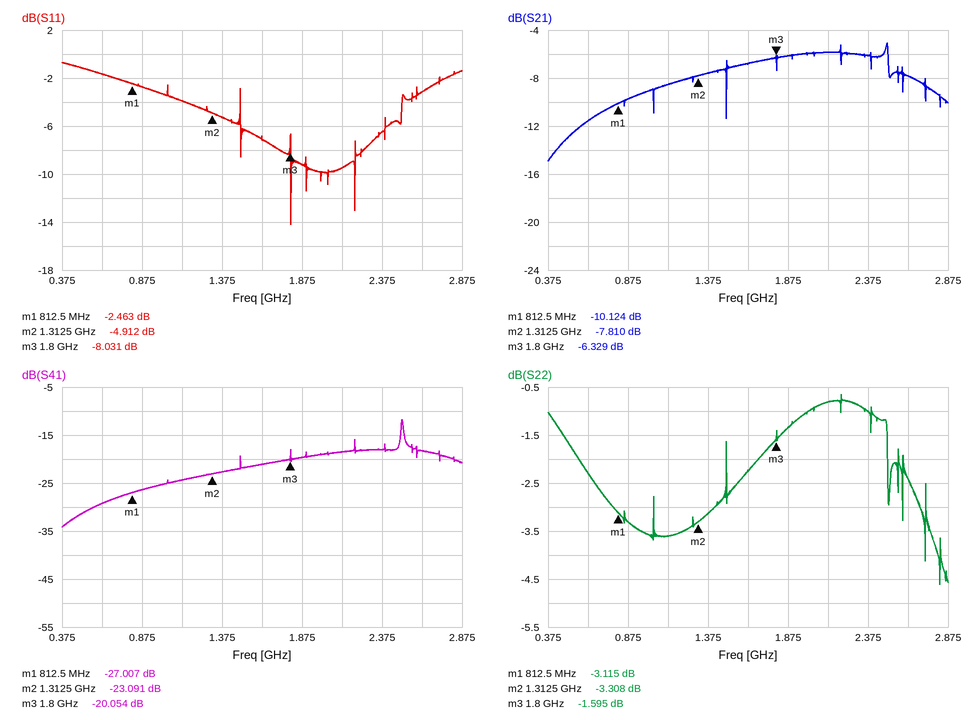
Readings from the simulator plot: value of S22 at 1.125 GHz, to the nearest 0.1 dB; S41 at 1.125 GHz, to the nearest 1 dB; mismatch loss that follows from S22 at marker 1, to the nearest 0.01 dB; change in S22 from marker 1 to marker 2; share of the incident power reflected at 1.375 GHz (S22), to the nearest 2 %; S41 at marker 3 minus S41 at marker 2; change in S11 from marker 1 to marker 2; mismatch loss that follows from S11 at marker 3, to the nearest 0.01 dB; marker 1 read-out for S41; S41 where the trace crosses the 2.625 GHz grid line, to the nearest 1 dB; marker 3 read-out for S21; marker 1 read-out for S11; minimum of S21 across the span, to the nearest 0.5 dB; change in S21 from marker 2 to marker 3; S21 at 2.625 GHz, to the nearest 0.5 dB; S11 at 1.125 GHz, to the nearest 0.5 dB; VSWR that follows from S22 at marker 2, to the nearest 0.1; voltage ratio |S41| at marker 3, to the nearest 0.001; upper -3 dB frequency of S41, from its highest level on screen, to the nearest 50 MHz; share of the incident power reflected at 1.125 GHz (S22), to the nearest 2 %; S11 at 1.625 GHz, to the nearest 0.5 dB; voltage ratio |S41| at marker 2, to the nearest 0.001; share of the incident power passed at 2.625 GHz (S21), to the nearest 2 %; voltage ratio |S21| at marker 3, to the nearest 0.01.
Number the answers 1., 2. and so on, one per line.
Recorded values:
1. -3.6 dB
2. -24 dB
3. 2.91 dB
4. -0.193 dB
5. 48 %
6. 3.037 dB
7. -2.449 dB
8. 0.74 dB
9. -27.007 dB
10. -18 dB
11. -6.329 dB
12. -2.463 dB
13. -15.0 dB
14. 1.481 dB
15. -8.0 dB
16. -4.0 dB
17. 5.3
18. 0.099
19. 2.50 GHz
20. 44 %
21. -7.0 dB
22. 0.070
23. 16 %
24. 0.48
